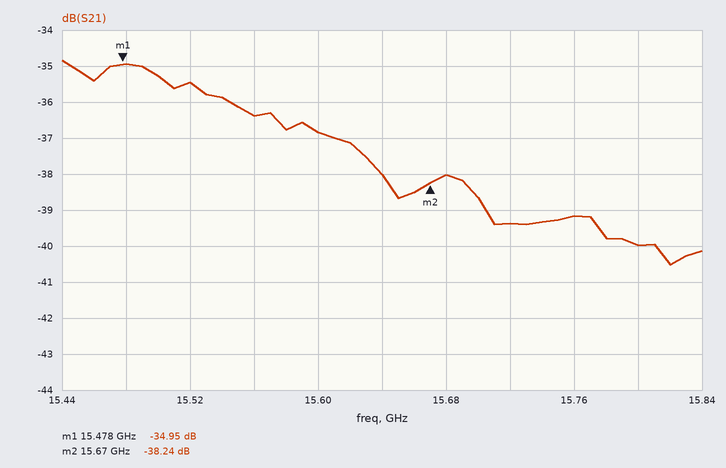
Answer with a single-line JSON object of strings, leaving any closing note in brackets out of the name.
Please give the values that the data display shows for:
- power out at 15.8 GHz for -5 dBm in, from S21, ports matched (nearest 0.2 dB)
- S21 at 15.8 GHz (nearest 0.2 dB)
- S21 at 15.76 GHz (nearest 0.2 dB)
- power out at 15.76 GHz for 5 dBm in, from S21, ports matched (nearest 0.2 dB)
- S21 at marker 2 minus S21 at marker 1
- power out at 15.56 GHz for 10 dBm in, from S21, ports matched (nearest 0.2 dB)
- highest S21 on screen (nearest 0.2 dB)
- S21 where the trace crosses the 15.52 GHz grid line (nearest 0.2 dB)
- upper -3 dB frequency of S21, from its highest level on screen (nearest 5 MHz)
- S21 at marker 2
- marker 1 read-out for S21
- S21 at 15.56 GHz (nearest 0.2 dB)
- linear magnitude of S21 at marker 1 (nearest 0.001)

{"power out at 15.8 GHz for -5 dBm in, from S21, ports matched": "-45.0 dBm", "S21 at 15.8 GHz": "-40.0 dB", "S21 at 15.76 GHz": "-39.2 dB", "power out at 15.76 GHz for 5 dBm in, from S21, ports matched": "-34.2 dBm", "S21 at marker 2 minus S21 at marker 1": "-3.29 dB", "power out at 15.56 GHz for 10 dBm in, from S21, ports matched": "-26.4 dBm", "highest S21 on screen": "-34.8 dB", "S21 where the trace crosses the 15.52 GHz grid line": "-35.4 dB", "upper -3 dB frequency of S21, from its highest level on screen": "15.635 GHz", "S21 at marker 2": "-38.24 dB", "marker 1 read-out for S21": "-34.95 dB", "S21 at 15.56 GHz": "-36.4 dB", "linear magnitude of S21 at marker 1": "0.018"}
